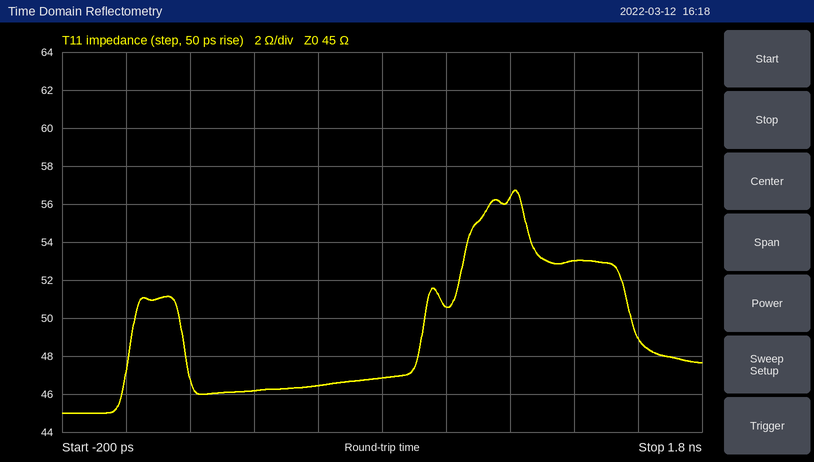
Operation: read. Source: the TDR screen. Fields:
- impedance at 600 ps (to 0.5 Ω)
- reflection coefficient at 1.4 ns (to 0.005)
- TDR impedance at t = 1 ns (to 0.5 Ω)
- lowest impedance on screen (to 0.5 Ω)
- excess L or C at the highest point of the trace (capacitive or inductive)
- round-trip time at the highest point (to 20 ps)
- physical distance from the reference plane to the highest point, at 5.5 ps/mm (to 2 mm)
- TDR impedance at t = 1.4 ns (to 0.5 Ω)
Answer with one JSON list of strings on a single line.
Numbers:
["46.5 Ω", "+0.080", "50.5 Ω", "45.0 Ω", "inductive", "1.22 ns", "110 mm", "53.0 Ω"]
